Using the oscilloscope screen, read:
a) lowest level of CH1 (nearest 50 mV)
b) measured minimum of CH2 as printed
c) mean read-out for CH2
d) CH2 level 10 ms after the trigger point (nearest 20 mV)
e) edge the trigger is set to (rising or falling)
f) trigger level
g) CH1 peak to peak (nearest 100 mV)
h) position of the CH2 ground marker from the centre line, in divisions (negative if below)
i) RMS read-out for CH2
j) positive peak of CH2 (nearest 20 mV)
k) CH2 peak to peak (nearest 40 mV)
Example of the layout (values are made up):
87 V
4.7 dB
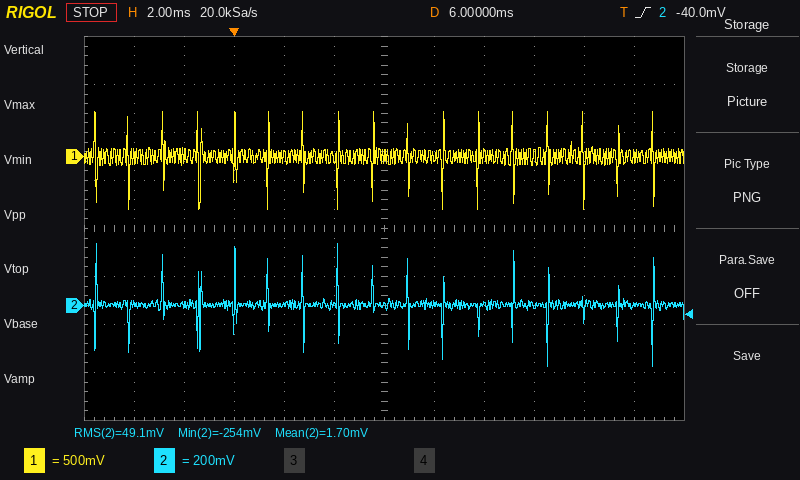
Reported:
-550 mV
-254 mV
1.70 mV
0 mV
rising
-40.0 mV
1.00 V
-1.6 div
49.1 mV
260 mV
520 mV
